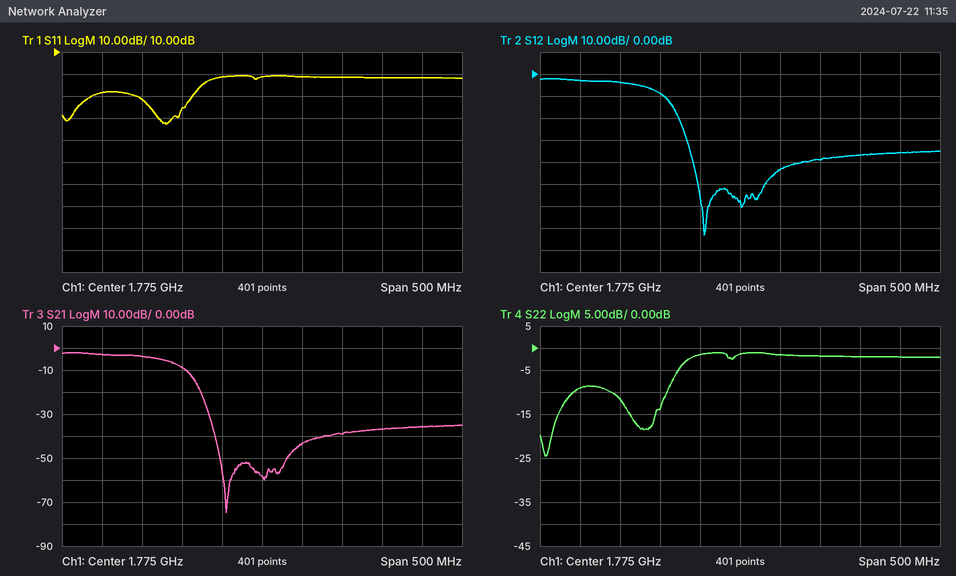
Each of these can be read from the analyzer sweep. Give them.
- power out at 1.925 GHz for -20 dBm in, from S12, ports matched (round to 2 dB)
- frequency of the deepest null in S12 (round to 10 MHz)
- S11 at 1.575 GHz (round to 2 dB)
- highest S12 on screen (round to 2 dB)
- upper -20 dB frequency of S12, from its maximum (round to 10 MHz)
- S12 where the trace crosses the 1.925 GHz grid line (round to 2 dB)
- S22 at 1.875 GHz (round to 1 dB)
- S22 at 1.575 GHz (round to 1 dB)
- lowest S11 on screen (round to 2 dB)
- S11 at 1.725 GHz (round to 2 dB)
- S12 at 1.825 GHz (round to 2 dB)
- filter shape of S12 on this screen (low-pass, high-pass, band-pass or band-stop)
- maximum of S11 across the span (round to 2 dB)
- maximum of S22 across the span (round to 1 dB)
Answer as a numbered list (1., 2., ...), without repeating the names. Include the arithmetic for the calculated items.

1. -20 dBm + (-36 dB) = -56 dBm
2. 1.73 GHz
3. -8 dB
4. -2 dB
5. 1.70 GHz
6. -36 dB
7. -2 dB
8. -9 dB
9. -22 dB
10. -2 dB
11. -44 dB
12. low-pass
13. 0 dB
14. -1 dB
